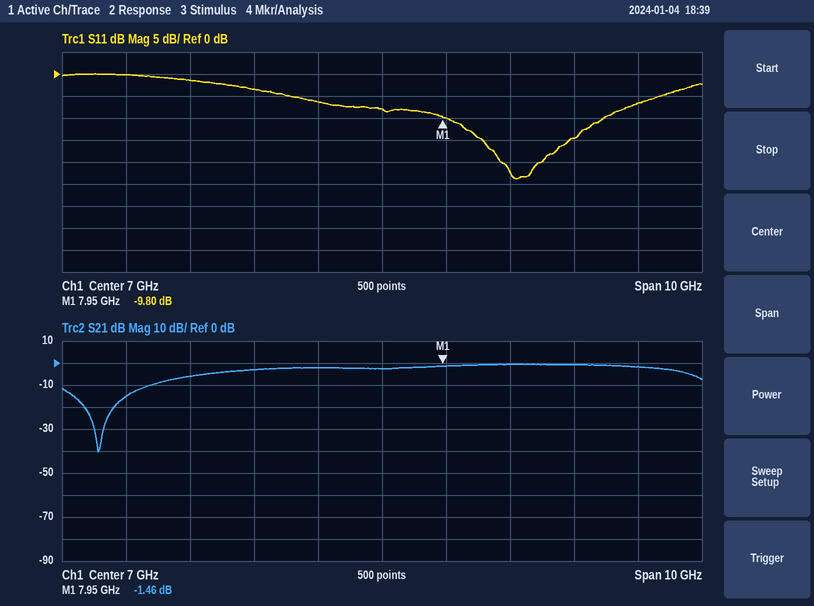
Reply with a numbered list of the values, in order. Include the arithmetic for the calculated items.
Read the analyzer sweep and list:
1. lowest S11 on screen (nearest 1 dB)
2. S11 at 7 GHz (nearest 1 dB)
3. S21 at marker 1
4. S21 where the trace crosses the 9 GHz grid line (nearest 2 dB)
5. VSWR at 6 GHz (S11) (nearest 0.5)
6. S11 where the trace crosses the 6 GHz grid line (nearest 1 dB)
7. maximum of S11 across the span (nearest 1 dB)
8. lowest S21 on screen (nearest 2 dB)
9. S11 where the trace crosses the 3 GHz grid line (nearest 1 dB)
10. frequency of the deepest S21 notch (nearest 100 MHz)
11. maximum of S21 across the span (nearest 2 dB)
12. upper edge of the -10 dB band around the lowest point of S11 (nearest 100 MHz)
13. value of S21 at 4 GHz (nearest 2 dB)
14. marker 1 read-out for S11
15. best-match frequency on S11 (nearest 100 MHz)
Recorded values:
1. -24 dB
2. -8 dB
3. -1.46 dB
4. 0 dB
5. |Γ| = 10^(-6/20) = 0.5012; VSWR = (1 + 0.5012)/(1 − 0.5012) ≈ 3.0
6. -6 dB
7. 0 dB
8. -40 dB
9. 0 dB
10. 2.6 GHz
11. 0 dB
12. 10.5 GHz
13. -6 dB
14. -9.80 dB
15. 9.1 GHz
